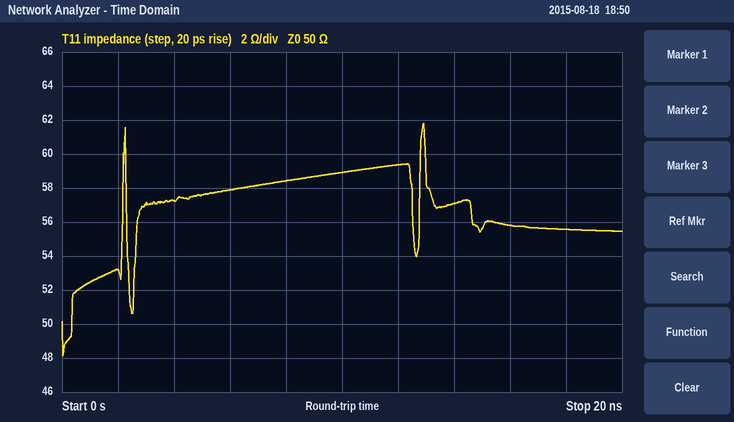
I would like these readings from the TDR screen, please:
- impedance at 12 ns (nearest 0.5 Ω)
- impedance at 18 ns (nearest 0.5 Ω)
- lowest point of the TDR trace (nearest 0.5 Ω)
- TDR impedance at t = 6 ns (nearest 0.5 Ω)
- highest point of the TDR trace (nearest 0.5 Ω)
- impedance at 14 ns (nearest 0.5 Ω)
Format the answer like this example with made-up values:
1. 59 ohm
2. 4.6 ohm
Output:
1. 59.5 Ω
2. 55.5 Ω
3. 48.0 Ω
4. 58.0 Ω
5. 62.0 Ω
6. 57.0 Ω
